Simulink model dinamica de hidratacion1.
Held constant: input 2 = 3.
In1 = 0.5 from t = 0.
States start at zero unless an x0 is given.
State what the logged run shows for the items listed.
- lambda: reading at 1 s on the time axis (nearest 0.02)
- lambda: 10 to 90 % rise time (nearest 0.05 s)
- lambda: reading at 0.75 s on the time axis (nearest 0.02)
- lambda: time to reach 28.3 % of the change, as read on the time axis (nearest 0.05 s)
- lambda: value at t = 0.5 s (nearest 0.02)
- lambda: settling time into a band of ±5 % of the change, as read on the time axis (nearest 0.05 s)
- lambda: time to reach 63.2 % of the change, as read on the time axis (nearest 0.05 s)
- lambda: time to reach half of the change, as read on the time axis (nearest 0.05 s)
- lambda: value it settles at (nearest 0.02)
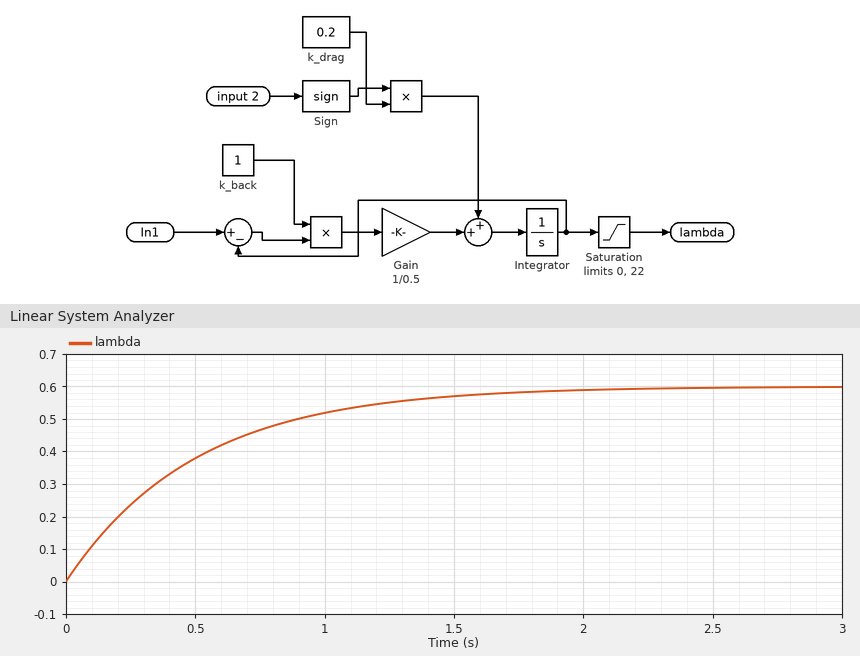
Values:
0.52
1.10 s
0.46
0.15 s
0.38
1.50 s
0.50 s
0.35 s
0.60
